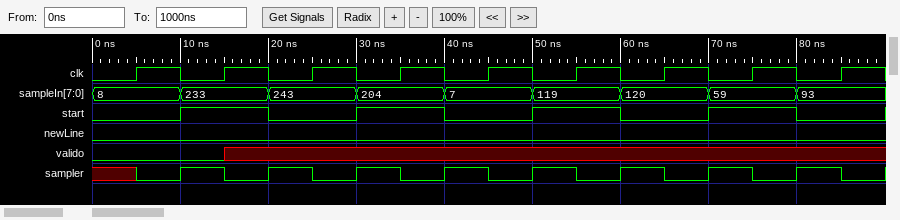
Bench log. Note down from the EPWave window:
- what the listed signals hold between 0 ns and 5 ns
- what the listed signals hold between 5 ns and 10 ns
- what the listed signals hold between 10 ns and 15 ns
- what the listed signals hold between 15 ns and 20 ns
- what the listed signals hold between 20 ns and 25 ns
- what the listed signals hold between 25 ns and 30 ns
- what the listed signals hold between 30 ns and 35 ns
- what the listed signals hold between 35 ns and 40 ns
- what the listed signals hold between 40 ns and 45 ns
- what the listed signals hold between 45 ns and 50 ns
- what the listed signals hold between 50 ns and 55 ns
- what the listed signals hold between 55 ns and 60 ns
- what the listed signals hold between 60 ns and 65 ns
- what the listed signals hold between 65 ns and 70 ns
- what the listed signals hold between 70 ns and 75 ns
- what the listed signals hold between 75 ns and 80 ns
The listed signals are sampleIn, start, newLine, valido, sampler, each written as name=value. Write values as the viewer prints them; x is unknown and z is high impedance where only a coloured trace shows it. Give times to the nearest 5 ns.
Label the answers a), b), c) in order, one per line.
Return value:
a) sampleIn=8, start=0, newLine=0, valido=0, sampler=x
b) sampleIn=8, start=0, newLine=0, valido=0, sampler=0
c) sampleIn=233, start=1, newLine=0, valido=0, sampler=1
d) sampleIn=233, start=1, newLine=0, valido=x, sampler=0
e) sampleIn=243, start=0, newLine=0, valido=x, sampler=1
f) sampleIn=243, start=0, newLine=0, valido=x, sampler=0
g) sampleIn=204, start=1, newLine=0, valido=x, sampler=1
h) sampleIn=204, start=1, newLine=0, valido=x, sampler=0
i) sampleIn=7, start=0, newLine=0, valido=x, sampler=1
j) sampleIn=7, start=0, newLine=0, valido=x, sampler=0
k) sampleIn=119, start=1, newLine=0, valido=x, sampler=1
l) sampleIn=119, start=1, newLine=0, valido=x, sampler=0
m) sampleIn=120, start=0, newLine=0, valido=x, sampler=1
n) sampleIn=120, start=0, newLine=0, valido=x, sampler=0
o) sampleIn=59, start=1, newLine=0, valido=x, sampler=1
p) sampleIn=59, start=1, newLine=0, valido=x, sampler=0
